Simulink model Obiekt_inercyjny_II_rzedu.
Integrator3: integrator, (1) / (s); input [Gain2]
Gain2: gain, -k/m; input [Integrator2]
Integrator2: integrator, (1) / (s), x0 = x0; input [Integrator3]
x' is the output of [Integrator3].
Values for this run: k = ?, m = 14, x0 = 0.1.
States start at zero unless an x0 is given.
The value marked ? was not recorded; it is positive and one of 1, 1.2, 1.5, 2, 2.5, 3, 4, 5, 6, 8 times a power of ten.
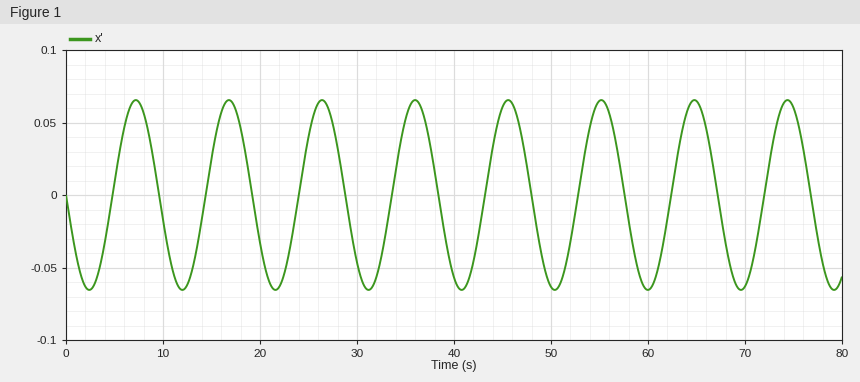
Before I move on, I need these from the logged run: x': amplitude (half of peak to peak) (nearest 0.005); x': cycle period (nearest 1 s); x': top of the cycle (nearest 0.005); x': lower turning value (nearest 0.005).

0.065
10 s
0.065
-0.065
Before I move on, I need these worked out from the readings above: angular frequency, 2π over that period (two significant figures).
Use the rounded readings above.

0.63 rad/s
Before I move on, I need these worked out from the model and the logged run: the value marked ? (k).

6
